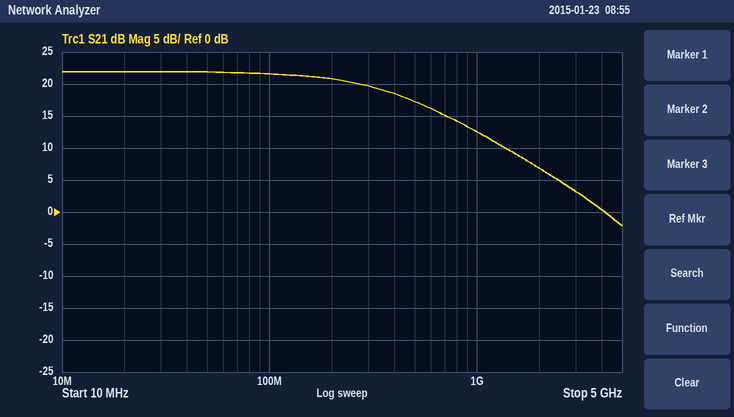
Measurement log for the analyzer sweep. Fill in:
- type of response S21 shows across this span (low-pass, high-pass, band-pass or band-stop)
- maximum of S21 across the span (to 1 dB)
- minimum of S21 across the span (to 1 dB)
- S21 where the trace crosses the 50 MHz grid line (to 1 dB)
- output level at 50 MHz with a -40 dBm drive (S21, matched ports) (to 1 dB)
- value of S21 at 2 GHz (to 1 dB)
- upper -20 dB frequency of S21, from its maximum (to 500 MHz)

low-pass
22 dB
-2 dB
22 dB
-18 dBm
7 dB
3.5 GHz
